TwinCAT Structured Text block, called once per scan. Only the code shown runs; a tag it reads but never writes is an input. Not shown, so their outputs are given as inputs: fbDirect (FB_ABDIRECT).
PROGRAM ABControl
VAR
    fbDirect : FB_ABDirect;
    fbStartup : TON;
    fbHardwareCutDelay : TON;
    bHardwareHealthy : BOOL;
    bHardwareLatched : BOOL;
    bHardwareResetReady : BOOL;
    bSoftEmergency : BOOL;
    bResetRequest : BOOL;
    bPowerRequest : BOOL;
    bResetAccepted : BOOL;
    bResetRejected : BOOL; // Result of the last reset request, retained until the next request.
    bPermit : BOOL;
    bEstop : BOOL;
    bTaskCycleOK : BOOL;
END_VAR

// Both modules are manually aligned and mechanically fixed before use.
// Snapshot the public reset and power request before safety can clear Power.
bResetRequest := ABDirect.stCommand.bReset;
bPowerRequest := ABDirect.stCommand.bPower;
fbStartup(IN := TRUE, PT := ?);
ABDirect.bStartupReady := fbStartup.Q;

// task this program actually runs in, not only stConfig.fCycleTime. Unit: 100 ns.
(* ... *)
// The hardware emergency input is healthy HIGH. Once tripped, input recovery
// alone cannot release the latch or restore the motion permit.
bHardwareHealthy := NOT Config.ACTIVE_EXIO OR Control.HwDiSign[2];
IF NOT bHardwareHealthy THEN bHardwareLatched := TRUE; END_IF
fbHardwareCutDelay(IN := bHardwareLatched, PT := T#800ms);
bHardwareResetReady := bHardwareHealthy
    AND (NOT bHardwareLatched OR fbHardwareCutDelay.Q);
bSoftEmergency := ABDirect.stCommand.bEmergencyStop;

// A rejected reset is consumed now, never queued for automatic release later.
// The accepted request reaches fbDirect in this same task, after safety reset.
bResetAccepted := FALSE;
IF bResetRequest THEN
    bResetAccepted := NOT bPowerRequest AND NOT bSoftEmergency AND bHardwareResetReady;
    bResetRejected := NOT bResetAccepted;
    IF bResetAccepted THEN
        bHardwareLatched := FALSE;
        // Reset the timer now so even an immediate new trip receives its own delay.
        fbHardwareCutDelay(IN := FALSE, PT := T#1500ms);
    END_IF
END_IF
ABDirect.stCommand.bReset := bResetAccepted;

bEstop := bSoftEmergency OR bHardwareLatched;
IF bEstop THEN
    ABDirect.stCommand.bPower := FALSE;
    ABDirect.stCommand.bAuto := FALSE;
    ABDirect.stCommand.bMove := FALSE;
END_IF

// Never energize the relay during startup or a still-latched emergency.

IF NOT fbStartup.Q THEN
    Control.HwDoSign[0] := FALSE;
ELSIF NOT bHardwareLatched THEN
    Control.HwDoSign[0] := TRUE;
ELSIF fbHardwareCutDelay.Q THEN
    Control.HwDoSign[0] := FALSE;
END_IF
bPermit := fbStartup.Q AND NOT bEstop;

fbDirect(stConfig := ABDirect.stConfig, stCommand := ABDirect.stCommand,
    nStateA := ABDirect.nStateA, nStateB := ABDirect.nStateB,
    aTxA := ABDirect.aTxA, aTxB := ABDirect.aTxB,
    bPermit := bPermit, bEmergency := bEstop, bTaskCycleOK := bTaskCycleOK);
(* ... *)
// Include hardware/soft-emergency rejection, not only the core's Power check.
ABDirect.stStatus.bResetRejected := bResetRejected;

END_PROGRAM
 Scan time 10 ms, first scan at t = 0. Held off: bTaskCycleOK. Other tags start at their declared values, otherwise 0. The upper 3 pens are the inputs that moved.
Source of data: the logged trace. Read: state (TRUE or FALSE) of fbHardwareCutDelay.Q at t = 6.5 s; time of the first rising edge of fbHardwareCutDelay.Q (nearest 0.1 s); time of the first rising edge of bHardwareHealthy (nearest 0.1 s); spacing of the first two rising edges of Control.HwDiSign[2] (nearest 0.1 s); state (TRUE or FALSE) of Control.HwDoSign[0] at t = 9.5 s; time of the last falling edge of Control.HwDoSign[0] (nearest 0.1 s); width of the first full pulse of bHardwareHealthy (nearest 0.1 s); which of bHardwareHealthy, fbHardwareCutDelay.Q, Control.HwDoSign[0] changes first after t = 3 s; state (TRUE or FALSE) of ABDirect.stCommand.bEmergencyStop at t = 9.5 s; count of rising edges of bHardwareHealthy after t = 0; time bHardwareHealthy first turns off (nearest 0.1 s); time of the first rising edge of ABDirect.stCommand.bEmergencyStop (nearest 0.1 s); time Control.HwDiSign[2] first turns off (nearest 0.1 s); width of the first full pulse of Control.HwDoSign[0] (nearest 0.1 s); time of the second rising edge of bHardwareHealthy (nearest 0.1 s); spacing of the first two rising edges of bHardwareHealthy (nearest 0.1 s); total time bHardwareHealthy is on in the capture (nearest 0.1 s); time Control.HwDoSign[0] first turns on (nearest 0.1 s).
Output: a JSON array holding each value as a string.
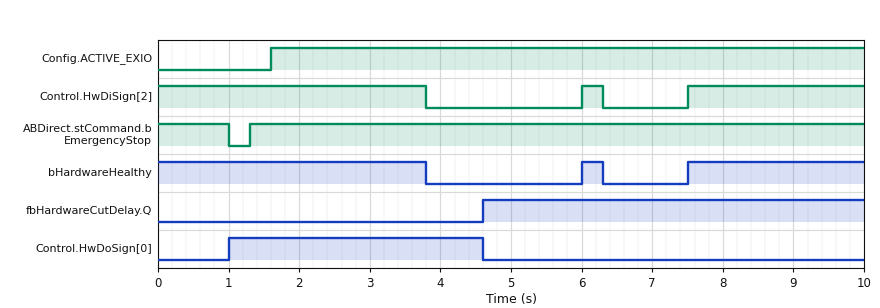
["TRUE", "4.6 s", "6.0 s", "1.5 s", "FALSE", "4.6 s", "0.3 s", "bHardwareHealthy", "TRUE", "2", "3.8 s", "1.3 s", "3.8 s", "3.6 s", "7.5 s", "1.5 s", "6.6 s", "1.0 s"]
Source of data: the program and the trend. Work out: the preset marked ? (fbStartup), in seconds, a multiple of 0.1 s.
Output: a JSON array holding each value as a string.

["1.0 s"]
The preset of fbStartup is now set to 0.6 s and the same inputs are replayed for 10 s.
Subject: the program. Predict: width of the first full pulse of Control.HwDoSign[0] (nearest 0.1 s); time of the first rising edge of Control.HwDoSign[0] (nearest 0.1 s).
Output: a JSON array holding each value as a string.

["4.0 s", "0.6 s"]
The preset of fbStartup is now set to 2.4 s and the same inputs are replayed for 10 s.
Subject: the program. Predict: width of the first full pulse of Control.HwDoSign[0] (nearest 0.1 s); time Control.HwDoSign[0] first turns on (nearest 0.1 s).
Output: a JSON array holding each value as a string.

["2.2 s", "2.4 s"]
